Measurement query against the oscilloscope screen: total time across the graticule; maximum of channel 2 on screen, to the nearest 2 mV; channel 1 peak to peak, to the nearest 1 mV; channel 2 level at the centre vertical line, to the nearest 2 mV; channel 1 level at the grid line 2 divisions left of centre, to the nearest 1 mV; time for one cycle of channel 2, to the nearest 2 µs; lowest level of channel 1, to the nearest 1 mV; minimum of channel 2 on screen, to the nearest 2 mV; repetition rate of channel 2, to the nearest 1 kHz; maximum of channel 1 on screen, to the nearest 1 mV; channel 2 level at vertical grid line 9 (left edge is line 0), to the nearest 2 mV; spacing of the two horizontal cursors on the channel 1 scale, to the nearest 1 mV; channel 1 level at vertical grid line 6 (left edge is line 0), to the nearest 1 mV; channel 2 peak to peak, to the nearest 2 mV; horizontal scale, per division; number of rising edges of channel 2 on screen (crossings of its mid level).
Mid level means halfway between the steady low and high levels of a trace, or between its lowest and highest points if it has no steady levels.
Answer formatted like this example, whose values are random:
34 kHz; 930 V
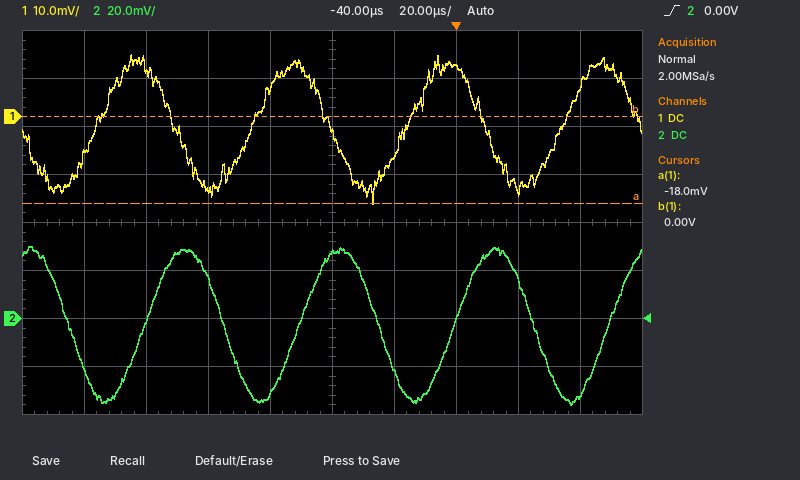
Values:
200 µs; 30 mV; 31 mV; 28 mV; -15 mV; 50 µs; -18 mV; -36 mV; 20 kHz; 13 mV; -32 mV; 18 mV; -8 mV; 66 mV; 20 µs; 4
